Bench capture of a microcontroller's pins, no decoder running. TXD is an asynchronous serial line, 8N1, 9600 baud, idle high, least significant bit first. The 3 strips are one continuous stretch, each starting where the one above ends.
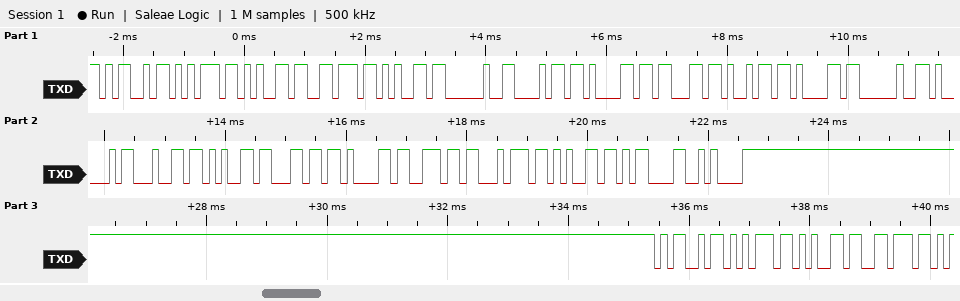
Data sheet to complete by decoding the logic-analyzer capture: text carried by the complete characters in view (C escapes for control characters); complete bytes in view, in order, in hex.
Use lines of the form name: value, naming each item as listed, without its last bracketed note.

text carried by the complete characters in view: "Mueve hacia Adelante\r\nMuev"
complete bytes in view, in order, in hex: 0x4D 0x75 0x65 0x76 0x65 0x20 0x68 0x61 0x63 0x69 0x61 0x20 0x41 0x64 0x65 0x6C 0x61 0x6E 0x74 0x65 0x0D 0x0A 0x4D 0x75 0x65 0x76
